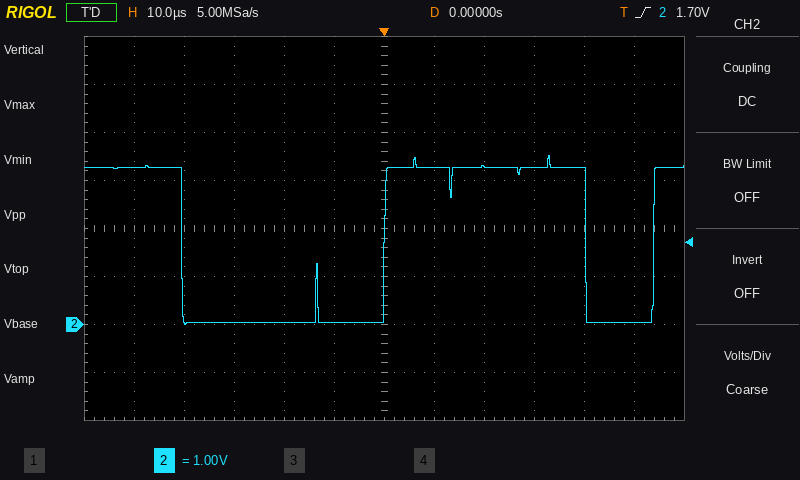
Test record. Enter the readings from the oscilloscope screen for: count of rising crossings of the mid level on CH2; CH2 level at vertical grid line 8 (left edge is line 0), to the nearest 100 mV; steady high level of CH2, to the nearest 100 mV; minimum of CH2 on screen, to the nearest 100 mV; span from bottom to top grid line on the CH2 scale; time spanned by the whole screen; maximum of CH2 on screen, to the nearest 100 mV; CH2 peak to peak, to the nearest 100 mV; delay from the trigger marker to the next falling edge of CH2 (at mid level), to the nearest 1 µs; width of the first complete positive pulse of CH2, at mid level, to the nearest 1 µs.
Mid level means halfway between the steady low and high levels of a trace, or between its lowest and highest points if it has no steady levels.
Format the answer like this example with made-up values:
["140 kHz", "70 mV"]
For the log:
["2", "3.3 V", "3.3 V", "0.0 V", "8 V", "120 µs", "3.5 V", "3.5 V", "40 µs", "40 µs"]
